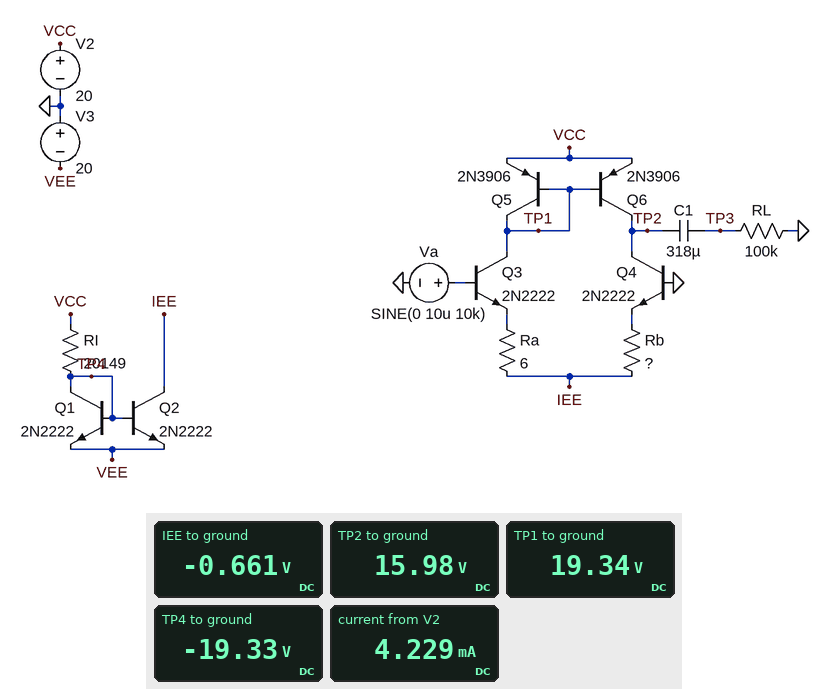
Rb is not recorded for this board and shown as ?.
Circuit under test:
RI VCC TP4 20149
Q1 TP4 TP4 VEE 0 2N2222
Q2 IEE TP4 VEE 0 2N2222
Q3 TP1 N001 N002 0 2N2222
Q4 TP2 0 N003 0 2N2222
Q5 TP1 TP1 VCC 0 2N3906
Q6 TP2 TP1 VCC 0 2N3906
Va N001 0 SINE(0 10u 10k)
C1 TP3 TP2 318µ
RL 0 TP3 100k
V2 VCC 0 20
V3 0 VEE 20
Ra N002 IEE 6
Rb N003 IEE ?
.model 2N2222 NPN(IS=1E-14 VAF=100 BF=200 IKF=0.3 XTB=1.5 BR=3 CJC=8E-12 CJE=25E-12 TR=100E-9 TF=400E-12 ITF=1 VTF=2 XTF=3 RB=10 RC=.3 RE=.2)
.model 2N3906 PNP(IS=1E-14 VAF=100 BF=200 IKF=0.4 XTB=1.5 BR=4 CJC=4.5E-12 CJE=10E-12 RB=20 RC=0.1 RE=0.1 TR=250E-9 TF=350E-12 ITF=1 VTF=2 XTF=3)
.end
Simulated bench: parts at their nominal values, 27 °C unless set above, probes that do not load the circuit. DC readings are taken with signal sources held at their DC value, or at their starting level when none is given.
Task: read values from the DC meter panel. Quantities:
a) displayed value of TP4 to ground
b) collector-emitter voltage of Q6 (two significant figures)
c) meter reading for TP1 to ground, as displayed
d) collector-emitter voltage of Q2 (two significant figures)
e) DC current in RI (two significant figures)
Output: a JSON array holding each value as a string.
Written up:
["-19.33 V", "-4.0 V", "19.34 V", "19 V", "2.0 mA"]
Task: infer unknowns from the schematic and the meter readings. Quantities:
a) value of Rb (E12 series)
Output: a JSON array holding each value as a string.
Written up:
["4.7 Ω"]
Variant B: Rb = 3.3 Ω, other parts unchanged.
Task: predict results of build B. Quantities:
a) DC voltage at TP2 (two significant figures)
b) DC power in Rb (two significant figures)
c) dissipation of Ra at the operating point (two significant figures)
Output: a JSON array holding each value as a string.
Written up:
["13 V", "4.5 µW", "7.4 µW"]
